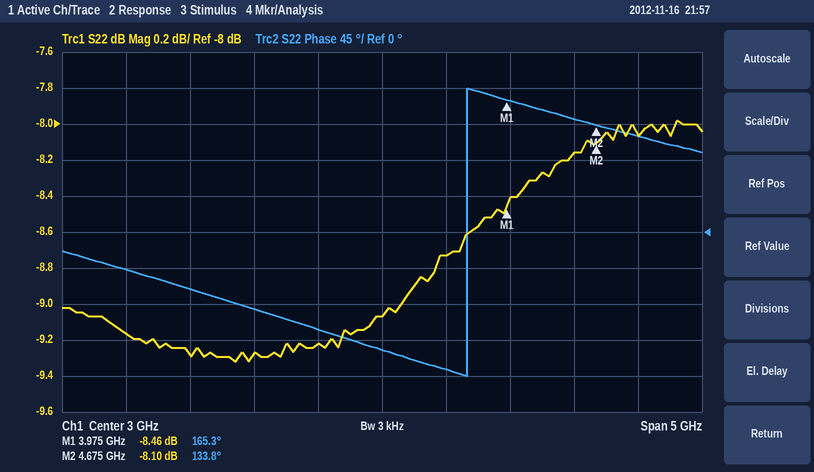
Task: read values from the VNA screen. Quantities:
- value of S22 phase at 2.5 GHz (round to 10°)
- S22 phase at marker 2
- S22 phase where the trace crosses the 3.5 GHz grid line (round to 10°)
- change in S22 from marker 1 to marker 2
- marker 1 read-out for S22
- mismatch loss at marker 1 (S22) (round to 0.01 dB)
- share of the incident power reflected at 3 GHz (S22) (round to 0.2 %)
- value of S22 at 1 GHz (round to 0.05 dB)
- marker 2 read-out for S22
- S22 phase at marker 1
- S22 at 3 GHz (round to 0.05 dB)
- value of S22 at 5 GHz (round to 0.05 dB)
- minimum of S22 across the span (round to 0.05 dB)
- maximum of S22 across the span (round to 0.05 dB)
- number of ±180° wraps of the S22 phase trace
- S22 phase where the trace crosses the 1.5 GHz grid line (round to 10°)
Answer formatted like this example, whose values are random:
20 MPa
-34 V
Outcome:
-120°
133.8°
-170°
0.36 dB
-8.46 dB
0.67 dB
12.4 %
-9.15 dB
-8.10 dB
165.3°
-9.05 dB
-8.05 dB
-9.30 dB
-8.00 dB
1
-70°
